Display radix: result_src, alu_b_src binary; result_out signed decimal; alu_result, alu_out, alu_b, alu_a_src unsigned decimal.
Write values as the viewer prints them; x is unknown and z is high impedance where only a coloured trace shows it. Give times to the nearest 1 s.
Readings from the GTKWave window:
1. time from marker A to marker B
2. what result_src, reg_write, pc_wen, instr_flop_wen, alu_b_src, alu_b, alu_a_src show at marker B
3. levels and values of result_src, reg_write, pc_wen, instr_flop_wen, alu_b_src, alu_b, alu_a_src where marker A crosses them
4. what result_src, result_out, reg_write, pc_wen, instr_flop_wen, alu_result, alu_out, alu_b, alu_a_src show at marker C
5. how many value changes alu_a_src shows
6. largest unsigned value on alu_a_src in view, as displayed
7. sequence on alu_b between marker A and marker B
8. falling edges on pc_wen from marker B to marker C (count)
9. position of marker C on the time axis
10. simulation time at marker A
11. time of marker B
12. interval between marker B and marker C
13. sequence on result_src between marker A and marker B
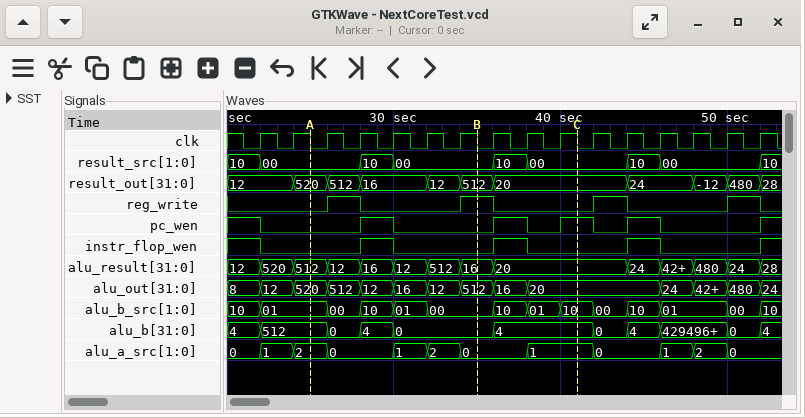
10 s
result_src=00, reg_write=1, pc_wen=0, instr_flop_wen=0, alu_b_src=00, alu_b=0, alu_a_src=0
result_src=00, reg_write=0, pc_wen=0, instr_flop_wen=0, alu_b_src=01, alu_b=512, alu_a_src=2
result_src=00, result_out=20, reg_write=0, pc_wen=1, instr_flop_wen=0, alu_result=20, alu_out=20, alu_b=4, alu_a_src=1
11
2
512, 0, 4, 0
1
41 s
25 s
35 s
6 s
00, 10, 00
